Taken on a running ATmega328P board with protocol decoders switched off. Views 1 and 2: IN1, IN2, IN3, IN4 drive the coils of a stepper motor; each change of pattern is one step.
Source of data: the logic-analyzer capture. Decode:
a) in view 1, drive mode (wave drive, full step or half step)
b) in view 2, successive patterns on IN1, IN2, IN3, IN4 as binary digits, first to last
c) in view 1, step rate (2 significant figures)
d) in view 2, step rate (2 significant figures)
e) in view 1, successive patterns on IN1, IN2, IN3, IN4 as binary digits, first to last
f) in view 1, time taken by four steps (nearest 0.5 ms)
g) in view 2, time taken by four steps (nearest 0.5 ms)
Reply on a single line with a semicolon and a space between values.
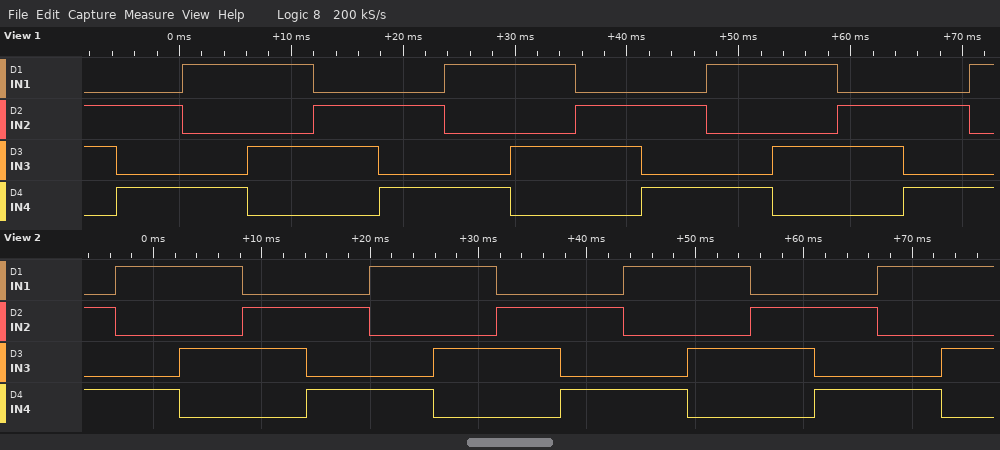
full step; 0101 1001 1010 0110 0101 1001 1010 0110 0101 1001 1010 0110 0101 1001 1010; 170 steps/s; 170 steps/s; 0110 0101 1001 1010 0110 0101 1001 1010 0110 0101 1001 1010 0110 0101 1001; 23.5 ms; 23.5 ms
